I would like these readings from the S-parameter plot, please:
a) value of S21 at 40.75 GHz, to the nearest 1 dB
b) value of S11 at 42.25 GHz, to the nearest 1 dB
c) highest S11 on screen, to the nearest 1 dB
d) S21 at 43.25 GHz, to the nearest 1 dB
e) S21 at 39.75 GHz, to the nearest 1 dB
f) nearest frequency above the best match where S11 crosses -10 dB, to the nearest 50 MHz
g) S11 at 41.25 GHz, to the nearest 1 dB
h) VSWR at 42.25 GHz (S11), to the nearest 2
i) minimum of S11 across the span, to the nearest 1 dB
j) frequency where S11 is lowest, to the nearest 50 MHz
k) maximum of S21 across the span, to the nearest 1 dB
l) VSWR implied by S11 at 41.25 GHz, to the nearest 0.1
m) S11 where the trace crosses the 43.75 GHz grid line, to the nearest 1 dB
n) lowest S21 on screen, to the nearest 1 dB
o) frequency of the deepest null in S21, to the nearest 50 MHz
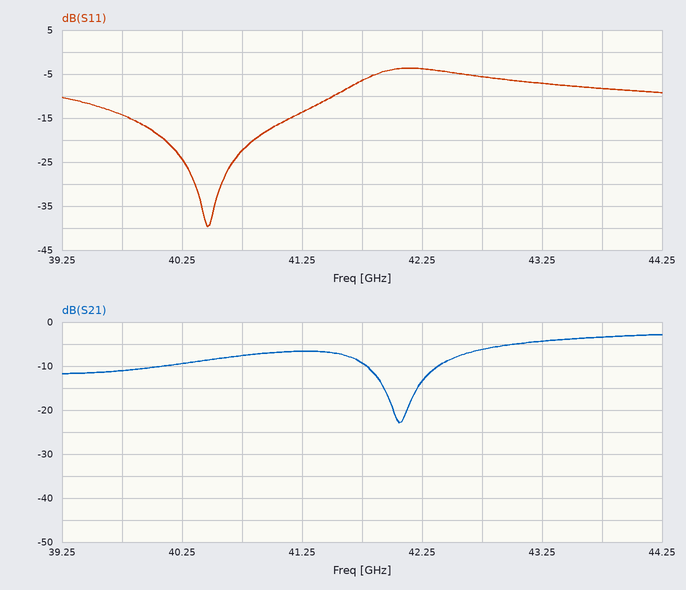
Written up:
-8 dB
-4 dB
-4 dB
-4 dB
-11 dB
41.50 GHz
-14 dB
4
-40 dB
40.45 GHz
-3 dB
1.5
-8 dB
-23 dB
42.05 GHz
